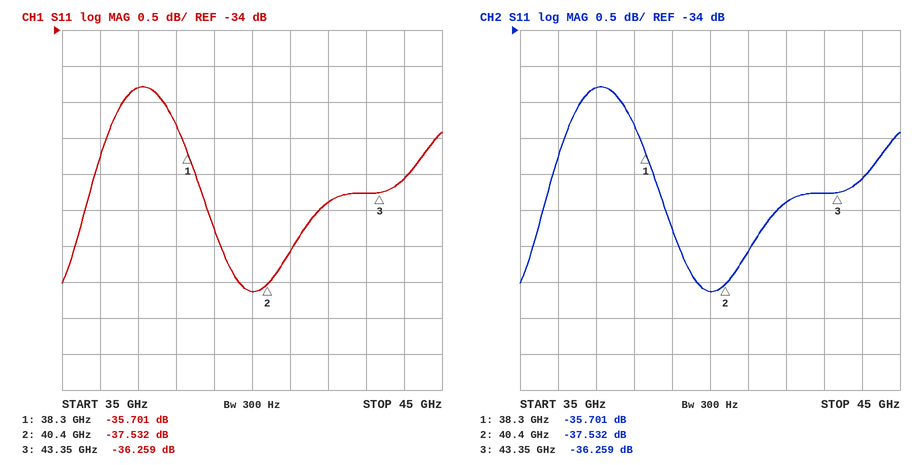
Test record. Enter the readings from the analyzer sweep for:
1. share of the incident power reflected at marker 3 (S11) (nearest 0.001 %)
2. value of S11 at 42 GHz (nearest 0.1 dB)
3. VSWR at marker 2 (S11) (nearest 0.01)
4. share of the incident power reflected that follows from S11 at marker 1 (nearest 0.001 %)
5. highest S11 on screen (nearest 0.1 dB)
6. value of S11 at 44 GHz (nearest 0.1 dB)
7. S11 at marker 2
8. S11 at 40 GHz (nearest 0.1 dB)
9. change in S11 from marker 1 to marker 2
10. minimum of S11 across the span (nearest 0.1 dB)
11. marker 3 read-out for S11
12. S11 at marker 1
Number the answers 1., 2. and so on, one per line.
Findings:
1. 0.024 %
2. -36.4 dB
3. 1.03
4. 0.027 %
5. -34.8 dB
6. -36.1 dB
7. -37.532 dB
8. -37.6 dB
9. -1.831 dB
10. -37.6 dB
11. -36.259 dB
12. -35.701 dB
